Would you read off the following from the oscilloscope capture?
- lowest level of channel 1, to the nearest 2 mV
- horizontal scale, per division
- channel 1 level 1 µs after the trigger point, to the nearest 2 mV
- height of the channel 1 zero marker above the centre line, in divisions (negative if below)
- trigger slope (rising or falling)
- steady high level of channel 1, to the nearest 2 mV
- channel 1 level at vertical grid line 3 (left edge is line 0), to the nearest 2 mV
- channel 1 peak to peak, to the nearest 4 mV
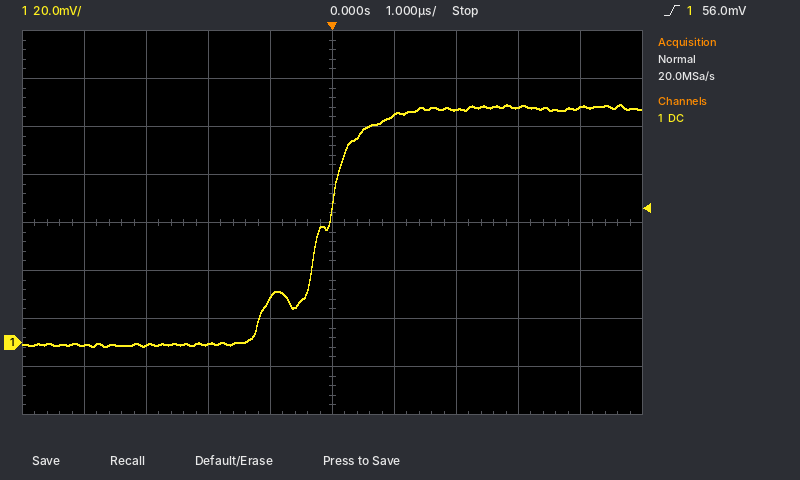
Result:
-2 mV
1 µs
94 mV
-2.5 div
rising
98 mV
0 mV
100 mV
